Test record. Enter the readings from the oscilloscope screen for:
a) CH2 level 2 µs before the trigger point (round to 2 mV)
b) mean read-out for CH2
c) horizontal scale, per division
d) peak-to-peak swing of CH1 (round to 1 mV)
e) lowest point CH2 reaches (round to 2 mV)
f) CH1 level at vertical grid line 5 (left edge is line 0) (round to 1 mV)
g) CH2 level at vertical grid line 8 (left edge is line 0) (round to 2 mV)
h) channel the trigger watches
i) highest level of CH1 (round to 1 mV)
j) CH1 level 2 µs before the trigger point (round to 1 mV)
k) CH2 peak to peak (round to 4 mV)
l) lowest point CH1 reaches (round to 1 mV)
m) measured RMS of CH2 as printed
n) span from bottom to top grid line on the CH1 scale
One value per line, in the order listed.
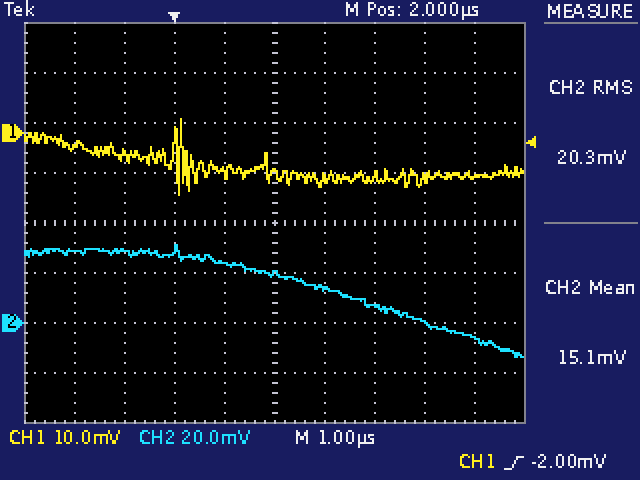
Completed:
28 mV
15.1 mV
1 µs
15 mV
-14 mV
-8 mV
0 mV
CH1
3 mV
-3 mV
44 mV
-12 mV
20.3 mV
80 mV
